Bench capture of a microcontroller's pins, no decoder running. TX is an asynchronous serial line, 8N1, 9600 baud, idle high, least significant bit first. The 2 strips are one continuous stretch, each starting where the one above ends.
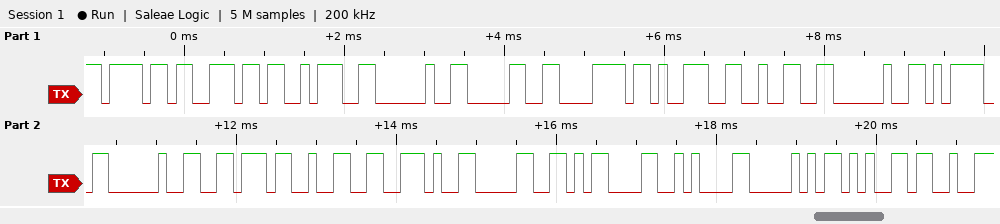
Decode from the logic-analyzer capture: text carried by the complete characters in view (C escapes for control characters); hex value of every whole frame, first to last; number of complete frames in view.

"on: 0x92 = v2.0\r\nPe"
6F 6E 3A 20 30 78 39 32 20 3D 20 76 32 2E 30 0D 0A 50 65
19
